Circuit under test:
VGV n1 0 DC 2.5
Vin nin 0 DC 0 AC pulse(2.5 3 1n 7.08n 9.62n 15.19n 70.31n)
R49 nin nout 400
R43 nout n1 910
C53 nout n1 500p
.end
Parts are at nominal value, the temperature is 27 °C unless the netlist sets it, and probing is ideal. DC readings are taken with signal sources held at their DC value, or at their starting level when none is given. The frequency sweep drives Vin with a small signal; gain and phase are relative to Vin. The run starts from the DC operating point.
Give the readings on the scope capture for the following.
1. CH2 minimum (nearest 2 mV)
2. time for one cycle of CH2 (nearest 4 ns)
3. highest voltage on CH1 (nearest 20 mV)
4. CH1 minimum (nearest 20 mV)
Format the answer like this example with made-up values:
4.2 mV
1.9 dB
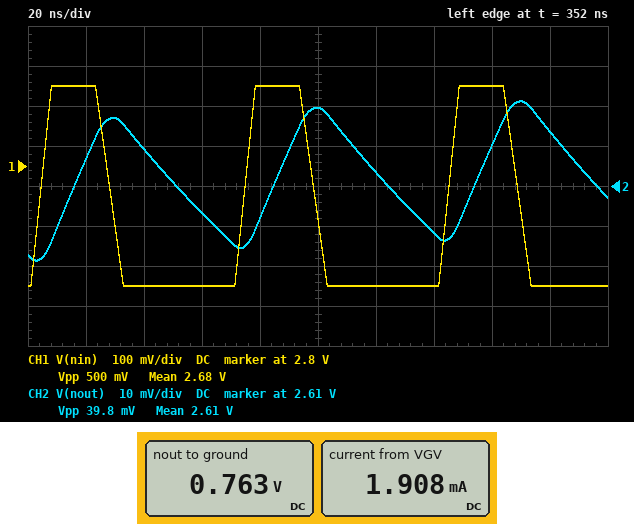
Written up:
2.592 V
68 ns
3.00 V
2.50 V
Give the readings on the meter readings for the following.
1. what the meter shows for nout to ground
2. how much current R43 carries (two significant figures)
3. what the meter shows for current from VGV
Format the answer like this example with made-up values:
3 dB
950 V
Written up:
0.763 V
1.9 mA
1.908 mA
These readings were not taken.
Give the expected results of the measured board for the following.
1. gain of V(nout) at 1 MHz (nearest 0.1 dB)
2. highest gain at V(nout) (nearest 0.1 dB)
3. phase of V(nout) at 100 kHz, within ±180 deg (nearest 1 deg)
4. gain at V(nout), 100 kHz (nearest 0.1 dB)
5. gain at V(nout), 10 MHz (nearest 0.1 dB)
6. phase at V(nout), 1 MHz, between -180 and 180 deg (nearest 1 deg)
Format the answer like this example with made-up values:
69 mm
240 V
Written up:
-5.6 dB
-3.2 dB
-5 deg
-3.2 dB
-22.0 dB
-41 deg
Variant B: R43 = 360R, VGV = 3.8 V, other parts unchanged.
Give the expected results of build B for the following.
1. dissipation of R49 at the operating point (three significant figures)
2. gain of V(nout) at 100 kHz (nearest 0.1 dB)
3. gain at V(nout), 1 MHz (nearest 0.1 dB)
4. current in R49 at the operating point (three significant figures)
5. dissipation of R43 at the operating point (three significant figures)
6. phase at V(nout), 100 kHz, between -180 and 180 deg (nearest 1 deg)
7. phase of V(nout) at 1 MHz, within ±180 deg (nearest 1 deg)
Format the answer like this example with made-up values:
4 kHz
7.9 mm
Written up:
10.0 mW
-6.5 dB
-7.8 dB
5.00 mA
9.00 mW
-3 deg
-31 deg
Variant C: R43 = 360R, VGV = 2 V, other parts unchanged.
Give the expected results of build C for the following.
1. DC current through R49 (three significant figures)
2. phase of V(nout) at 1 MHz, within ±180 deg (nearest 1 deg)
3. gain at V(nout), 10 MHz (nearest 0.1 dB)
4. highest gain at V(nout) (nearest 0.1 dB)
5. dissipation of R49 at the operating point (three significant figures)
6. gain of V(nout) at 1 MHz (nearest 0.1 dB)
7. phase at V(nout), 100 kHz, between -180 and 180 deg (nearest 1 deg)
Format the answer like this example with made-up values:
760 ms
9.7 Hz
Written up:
2.63 mA
-31 deg
-22.1 dB
-6.5 dB
2.77 mW
-7.8 dB
-3 deg
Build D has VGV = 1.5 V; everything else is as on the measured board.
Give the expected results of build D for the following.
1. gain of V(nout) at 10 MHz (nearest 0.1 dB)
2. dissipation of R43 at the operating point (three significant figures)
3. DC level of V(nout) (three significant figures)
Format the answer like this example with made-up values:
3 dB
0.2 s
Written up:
-22.0 dB
1.19 mW
458 mV
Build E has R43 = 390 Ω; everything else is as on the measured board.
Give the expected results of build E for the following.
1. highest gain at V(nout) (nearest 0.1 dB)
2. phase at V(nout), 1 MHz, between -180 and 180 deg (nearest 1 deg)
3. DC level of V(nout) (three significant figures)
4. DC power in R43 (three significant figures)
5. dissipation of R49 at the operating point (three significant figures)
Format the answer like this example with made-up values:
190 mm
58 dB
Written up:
-6.1 dB
-32 deg
1.27 V
3.91 mW
4.01 mW
